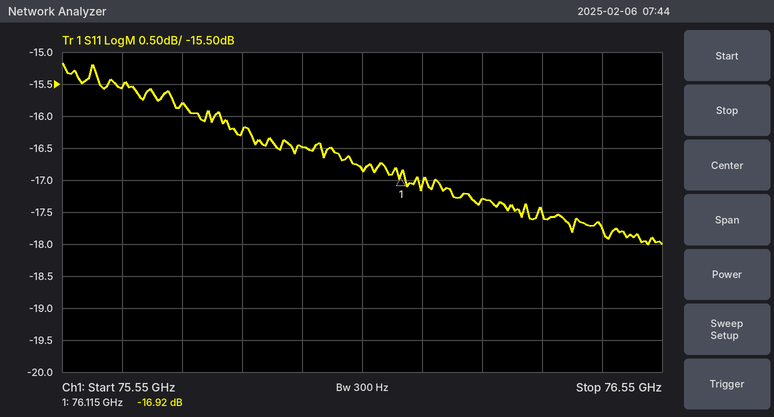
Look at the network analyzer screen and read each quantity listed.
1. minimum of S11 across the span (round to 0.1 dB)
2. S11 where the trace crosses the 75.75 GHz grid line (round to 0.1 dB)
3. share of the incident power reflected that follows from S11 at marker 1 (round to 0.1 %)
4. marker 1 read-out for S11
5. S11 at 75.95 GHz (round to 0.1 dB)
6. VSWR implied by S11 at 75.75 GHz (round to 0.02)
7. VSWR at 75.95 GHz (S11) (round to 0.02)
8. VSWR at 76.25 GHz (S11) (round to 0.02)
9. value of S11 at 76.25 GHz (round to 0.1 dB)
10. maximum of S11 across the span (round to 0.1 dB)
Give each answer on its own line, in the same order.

-18.0 dB
-15.8 dB
2.0 %
-16.92 dB
-16.5 dB
1.38
1.36
1.32
-17.3 dB
-15.2 dB
